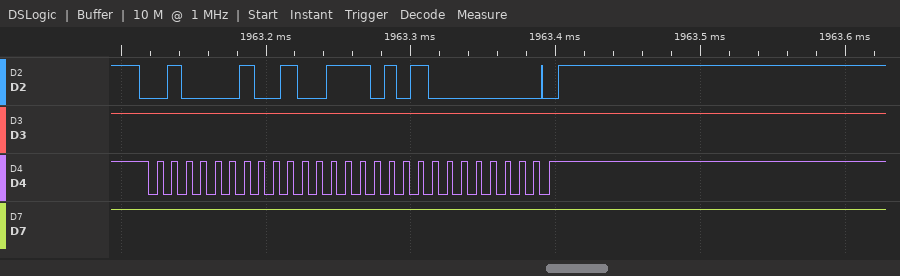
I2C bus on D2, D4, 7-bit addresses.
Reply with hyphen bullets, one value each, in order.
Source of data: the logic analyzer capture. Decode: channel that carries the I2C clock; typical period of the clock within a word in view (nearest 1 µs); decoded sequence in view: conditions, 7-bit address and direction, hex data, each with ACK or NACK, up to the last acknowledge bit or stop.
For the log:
- D4
- 10 µs
- start, address 21 write ACK, 9D ACK, 80 ACK, stop
